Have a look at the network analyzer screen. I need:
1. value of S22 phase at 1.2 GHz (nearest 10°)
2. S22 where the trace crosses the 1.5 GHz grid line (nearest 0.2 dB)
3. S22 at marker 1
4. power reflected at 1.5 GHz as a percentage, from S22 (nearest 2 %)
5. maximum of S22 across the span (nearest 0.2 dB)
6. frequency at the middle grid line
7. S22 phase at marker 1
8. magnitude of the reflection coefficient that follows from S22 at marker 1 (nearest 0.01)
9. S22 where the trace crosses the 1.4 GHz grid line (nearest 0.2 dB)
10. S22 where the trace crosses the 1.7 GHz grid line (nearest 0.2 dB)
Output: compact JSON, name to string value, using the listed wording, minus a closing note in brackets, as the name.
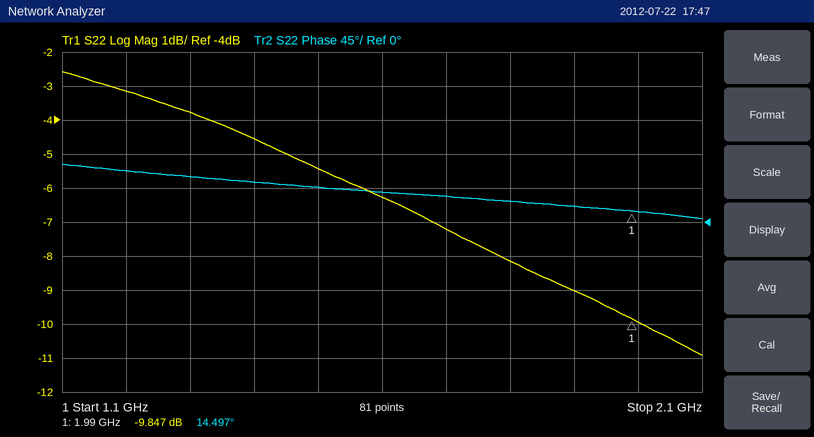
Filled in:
{"value of S22 phase at 1.2 GHz": "70°", "S22 where the trace crosses the 1.5 GHz grid line": "-5.4 dB", "S22 at marker 1": "-9.847 dB", "power reflected at 1.5 GHz as a percentage, from S22": "28 %", "maximum of S22 across the span": "-2.6 dB", "frequency at the middle grid line": "1.6 GHz", "S22 phase at marker 1": "14.497°", "magnitude of the reflection coefficient that follows from S22 at marker 1": "0.32", "S22 where the trace crosses the 1.4 GHz grid line": "-4.6 dB", "S22 where the trace crosses the 1.7 GHz grid line": "-7.2 dB"}
